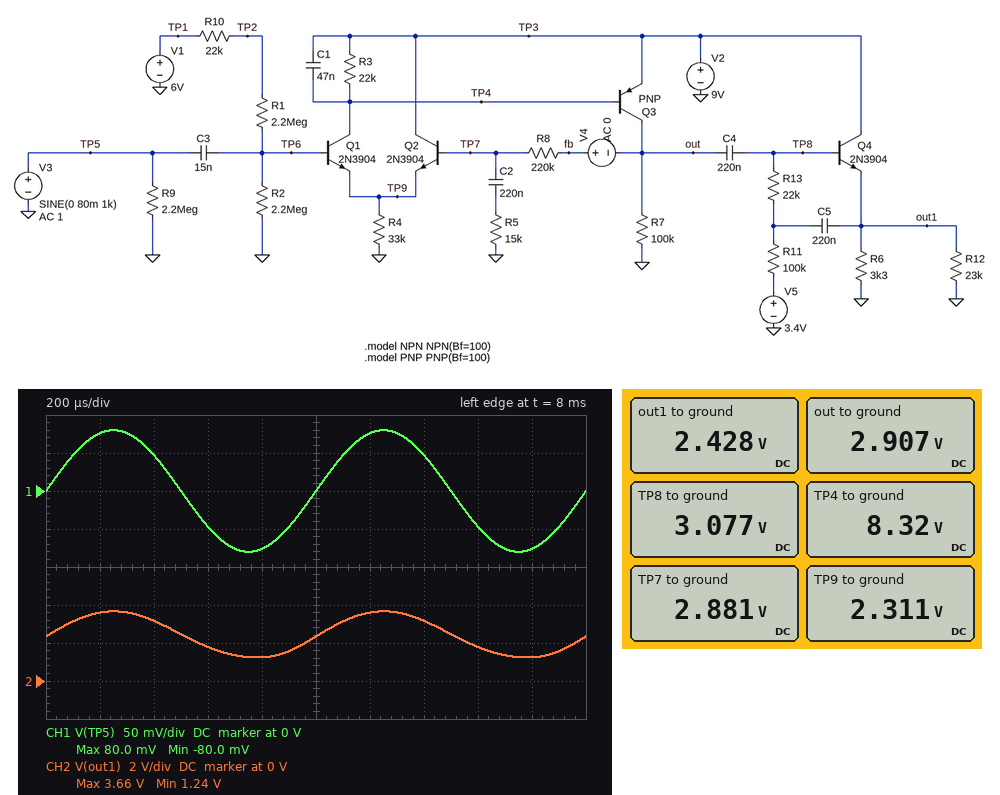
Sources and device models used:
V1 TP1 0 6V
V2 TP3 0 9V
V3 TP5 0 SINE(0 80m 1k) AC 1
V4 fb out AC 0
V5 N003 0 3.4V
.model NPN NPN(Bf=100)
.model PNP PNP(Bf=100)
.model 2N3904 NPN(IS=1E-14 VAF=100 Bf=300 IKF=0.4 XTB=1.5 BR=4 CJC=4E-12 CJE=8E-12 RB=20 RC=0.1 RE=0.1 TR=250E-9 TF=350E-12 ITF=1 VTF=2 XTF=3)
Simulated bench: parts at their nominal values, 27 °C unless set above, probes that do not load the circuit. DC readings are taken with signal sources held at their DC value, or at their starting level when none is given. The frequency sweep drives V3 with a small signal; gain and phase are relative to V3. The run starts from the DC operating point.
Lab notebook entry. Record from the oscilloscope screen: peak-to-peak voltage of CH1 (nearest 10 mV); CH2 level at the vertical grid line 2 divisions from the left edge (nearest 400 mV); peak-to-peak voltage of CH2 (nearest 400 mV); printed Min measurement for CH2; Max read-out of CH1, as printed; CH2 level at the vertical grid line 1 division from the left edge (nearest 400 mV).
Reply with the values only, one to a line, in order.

160 mV
3.2 V
2.4 V
1.24 V
80.0 mV
3.6 V
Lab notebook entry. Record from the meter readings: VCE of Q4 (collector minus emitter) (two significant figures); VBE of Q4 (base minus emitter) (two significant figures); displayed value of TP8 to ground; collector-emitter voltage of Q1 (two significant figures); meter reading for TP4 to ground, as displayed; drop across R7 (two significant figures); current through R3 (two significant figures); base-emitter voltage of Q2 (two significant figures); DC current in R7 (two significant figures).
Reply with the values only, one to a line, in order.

6.6 V
650 mV
3.077 V
6.0 V
8.32 V
2.9 V
31 µA
570 mV
29 µA
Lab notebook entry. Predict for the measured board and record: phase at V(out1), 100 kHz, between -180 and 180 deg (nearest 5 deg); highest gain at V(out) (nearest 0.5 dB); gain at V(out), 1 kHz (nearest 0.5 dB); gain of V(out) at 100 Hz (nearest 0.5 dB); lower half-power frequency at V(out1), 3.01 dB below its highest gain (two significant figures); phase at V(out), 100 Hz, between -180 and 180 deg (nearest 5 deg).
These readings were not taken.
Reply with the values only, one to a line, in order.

-90 deg
24.0 dB
24.0 dB
23.0 dB
44 Hz
30 deg
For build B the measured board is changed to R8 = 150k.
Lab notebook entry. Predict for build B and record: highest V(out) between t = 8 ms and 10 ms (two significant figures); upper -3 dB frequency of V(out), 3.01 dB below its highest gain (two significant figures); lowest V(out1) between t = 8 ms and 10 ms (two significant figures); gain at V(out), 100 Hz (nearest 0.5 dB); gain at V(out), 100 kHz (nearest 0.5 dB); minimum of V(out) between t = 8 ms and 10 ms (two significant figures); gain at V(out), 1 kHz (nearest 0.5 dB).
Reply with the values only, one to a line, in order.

3.8 V
13 kHz
1.6 V
20.0 dB
3.0 dB
2.0 V
21.0 dB
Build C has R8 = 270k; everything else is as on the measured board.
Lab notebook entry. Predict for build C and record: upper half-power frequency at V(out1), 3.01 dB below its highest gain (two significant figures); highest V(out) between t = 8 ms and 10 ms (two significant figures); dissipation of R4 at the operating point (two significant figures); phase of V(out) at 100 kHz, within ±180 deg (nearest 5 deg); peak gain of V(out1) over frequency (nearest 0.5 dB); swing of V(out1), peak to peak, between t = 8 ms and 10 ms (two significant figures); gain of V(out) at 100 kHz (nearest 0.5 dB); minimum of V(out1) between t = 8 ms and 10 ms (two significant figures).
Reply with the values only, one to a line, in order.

8.9 kHz
4.4 V
160 µW
-95 deg
25.5 dB
2.9 V
4.5 dB
1.0 V
